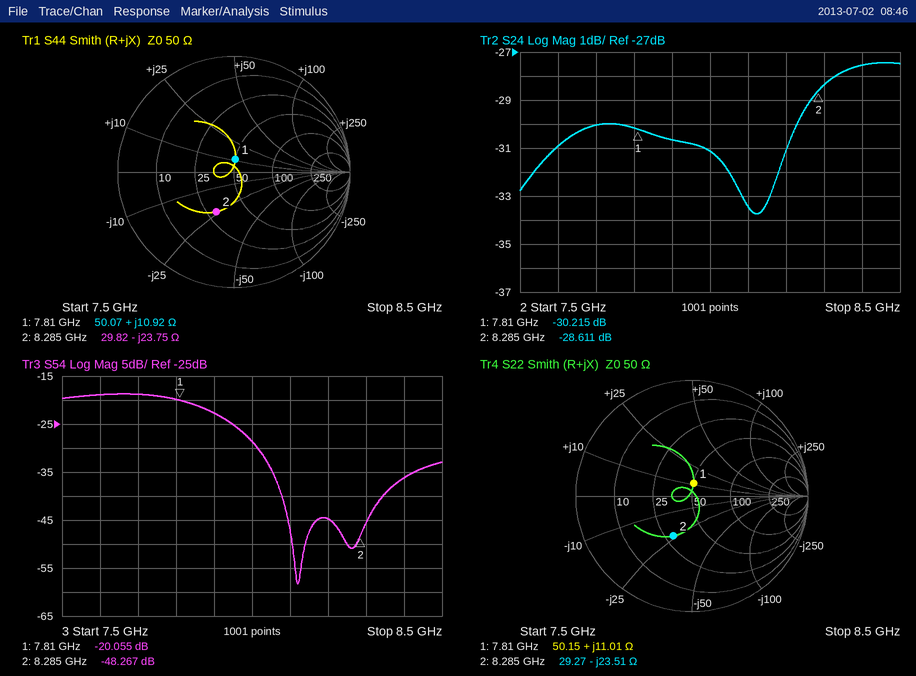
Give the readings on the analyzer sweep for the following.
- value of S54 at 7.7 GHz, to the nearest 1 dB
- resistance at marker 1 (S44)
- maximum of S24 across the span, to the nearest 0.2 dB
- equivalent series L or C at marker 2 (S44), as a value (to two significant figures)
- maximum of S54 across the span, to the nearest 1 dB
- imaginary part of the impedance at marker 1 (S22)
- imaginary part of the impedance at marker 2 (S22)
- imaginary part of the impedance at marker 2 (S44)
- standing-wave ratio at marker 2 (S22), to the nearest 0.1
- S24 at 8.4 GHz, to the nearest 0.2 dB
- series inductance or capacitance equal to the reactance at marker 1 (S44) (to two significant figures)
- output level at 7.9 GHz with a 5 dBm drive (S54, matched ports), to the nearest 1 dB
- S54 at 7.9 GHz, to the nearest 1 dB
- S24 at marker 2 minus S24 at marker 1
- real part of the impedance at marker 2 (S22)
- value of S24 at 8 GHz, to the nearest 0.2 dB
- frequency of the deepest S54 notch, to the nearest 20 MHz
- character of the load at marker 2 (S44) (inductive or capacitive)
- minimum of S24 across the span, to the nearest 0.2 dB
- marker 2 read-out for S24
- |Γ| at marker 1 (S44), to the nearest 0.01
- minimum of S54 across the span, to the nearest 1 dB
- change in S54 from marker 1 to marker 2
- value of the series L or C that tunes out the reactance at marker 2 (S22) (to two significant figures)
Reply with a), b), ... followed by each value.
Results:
a) -19 dB
b) 50.07 Ω
c) -27.4 dB
d) 810 fF
e) -19 dB
f) +11.01 Ω
g) -23.51 Ω
h) -23.75 Ω
i) 2.2
j) -27.6 dB
k) 220 pH
l) -18 dBm
m) -23 dB
n) 1.604 dB
o) 29.27 Ω
p) -31.2 dB
q) 8.12 GHz
r) capacitive
s) -33.8 dB
t) -28.611 dB
u) 0.11
v) -58 dB
w) -28.212 dB
x) 450 pH
